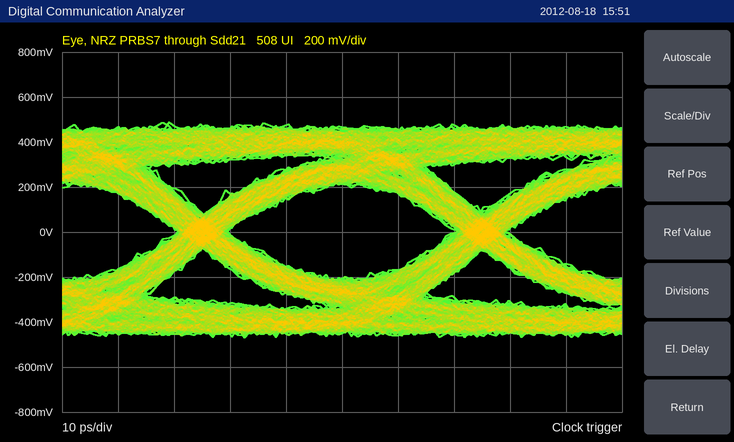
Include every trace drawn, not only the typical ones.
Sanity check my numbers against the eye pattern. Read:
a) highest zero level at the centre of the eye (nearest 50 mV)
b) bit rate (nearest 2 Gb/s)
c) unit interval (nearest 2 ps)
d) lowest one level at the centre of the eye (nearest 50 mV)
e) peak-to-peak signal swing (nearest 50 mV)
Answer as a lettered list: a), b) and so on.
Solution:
a) -200 mV
b) 20 Gb/s
c) 50 ps
d) 200 mV
e) 950 mV
